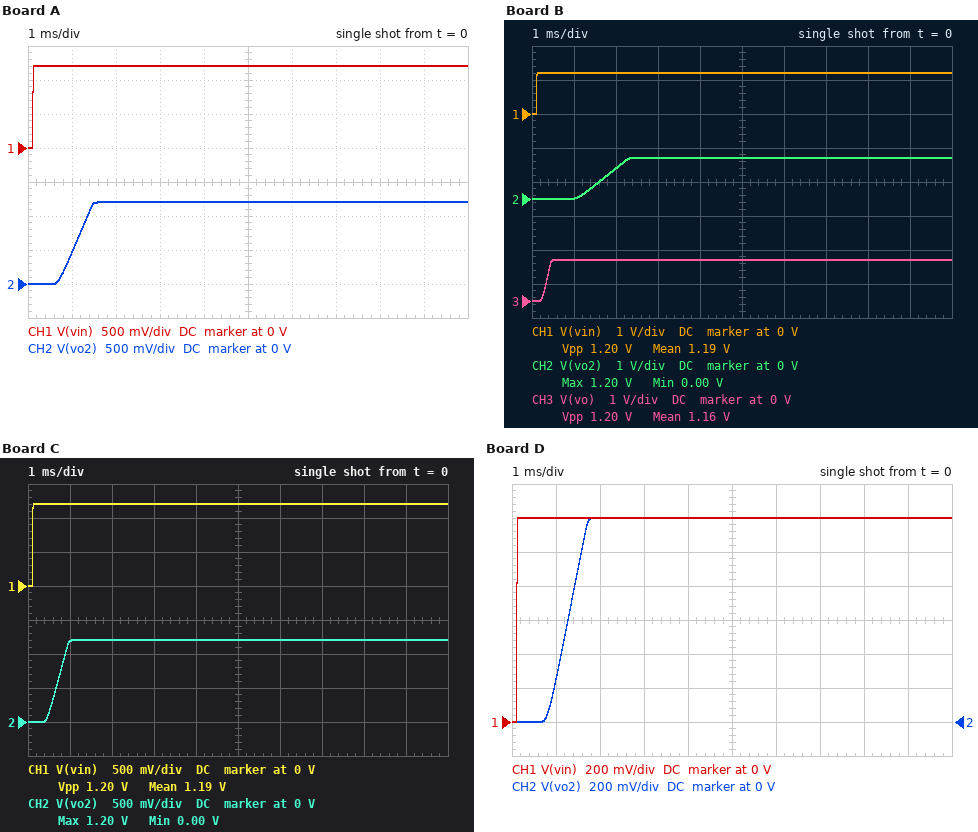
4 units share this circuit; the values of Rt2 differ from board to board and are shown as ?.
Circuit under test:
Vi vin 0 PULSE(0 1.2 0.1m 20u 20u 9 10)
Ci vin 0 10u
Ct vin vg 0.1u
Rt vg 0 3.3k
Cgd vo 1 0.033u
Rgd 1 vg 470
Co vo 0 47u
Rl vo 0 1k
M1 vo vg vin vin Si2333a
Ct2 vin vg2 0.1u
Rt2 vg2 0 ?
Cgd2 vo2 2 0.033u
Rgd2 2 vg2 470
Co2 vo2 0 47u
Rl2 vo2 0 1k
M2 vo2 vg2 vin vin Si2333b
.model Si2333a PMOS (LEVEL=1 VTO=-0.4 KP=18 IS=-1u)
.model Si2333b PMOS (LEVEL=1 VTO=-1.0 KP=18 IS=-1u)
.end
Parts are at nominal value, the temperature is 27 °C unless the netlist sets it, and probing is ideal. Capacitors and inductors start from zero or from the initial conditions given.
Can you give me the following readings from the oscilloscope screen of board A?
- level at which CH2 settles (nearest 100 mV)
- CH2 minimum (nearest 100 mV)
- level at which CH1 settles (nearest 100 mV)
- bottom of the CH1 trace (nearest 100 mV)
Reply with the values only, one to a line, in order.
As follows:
1.2 V
0 V
1.2 V
0 V
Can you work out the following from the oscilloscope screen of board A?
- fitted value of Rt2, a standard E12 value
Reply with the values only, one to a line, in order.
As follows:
2.2 kΩ
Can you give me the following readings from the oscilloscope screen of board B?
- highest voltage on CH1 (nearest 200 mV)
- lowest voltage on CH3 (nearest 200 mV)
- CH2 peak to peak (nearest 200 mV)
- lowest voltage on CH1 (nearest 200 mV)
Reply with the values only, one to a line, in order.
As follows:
1.2 V
0 V
1.2 V
0 V
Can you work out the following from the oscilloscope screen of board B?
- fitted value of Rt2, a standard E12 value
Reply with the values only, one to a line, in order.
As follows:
3.9 kΩ
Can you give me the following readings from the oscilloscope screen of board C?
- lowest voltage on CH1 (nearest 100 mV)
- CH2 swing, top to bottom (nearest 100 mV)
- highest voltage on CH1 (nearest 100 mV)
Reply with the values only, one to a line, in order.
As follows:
0 V
1.2 V
1.2 V
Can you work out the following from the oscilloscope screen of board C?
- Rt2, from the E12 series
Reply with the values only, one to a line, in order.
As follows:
1.2 kΩ
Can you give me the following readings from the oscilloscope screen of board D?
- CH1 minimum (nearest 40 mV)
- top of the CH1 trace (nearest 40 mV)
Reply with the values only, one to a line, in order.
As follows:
0 V
1.20 V
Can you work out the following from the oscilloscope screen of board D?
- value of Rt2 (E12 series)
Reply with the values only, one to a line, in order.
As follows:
2.7 kΩ
